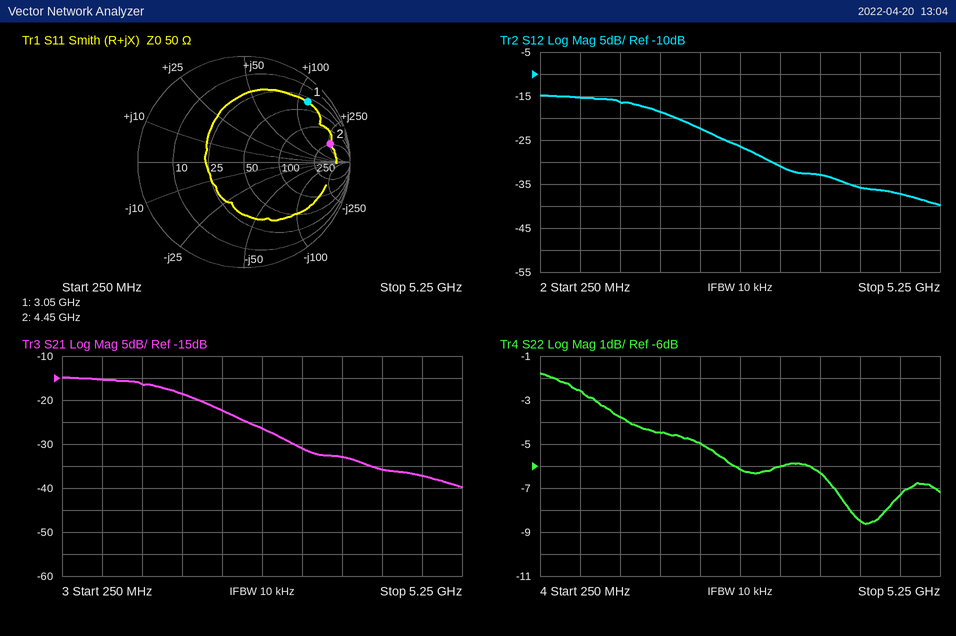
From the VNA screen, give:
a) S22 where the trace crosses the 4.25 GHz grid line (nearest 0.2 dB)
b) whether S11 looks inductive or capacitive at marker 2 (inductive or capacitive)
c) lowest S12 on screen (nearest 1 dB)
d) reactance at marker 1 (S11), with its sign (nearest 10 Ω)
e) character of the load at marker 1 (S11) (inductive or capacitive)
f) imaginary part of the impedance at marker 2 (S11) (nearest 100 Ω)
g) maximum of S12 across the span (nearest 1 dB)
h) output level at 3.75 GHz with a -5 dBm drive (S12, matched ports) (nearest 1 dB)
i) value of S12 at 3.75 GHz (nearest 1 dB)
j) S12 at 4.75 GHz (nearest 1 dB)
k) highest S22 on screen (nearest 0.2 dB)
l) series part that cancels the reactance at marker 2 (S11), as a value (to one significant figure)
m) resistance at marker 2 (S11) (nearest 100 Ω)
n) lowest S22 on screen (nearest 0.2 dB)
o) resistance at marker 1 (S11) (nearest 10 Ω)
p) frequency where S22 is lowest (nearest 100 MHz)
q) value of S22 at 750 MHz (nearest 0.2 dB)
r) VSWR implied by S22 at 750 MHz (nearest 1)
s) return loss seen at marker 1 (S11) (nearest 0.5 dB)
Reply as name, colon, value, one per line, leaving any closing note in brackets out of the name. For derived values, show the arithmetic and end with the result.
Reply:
S22 where the trace crosses the 4.25 GHz grid line: -8.4 dB
whether S11 looks inductive or capacitive at marker 2: inductive
lowest S12 on screen: -40 dB
reactance at marker 1 (S11), with its sign: +120 Ω
character of the load at marker 1 (S11): inductive
imaginary part of the impedance at marker 2 (S11): +300 Ω
maximum of S12 across the span: -15 dB
output level at 3.75 GHz with a -5 dBm drive (S12, matched ports): -5 dBm + (-33 dB) = -38 dBm
value of S12 at 3.75 GHz: -33 dB
S12 at 4.75 GHz: -37 dB
highest S22 on screen: -1.8 dB
series part that cancels the reactance at marker 2 (S11), as a value: C = 1/(2π × 4.45 GHz × 300 Ω) ≈ 119 fF, so 100 fF to one significant figure
resistance at marker 2 (S11): 200 Ω
lowest S22 on screen: -8.6 dB
resistance at marker 1 (S11): 30 Ω
frequency where S22 is lowest: 4.3 GHz
value of S22 at 750 MHz: -2.6 dB
VSWR implied by S22 at 750 MHz: |Γ| = 10^(-2.6/20) = 0.7413; VSWR = (1 + 0.7413)/(1 − 0.7413) ≈ 7
return loss seen at marker 1 (S11): 1.5 dB
